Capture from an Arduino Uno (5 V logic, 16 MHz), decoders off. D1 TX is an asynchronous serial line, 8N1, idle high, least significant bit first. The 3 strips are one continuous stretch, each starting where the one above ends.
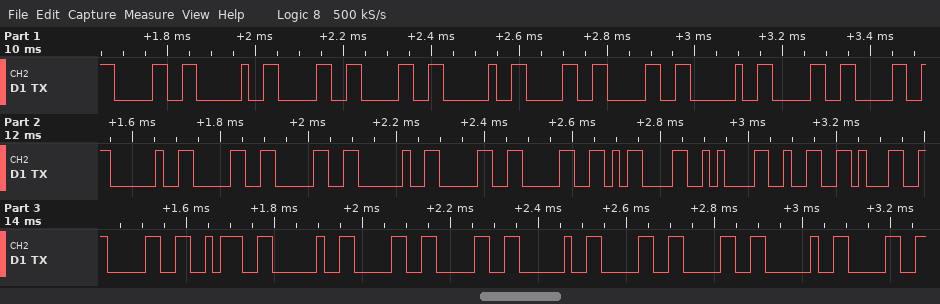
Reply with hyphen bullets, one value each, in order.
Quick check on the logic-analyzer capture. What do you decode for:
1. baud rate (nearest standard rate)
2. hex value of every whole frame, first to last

- 57600 baud
- 0x30 0x20 0x30 0x30 0x20 0x30 0x30 0x20 0x30 0x30 0x20 0x30 0x30 0x20 0x30 0x30 0x0D 0x0A 0x32 0x31 0x30 0x3A 0x20 0x30 0x30 0x20 0x30 0x30 0x20 0x30
